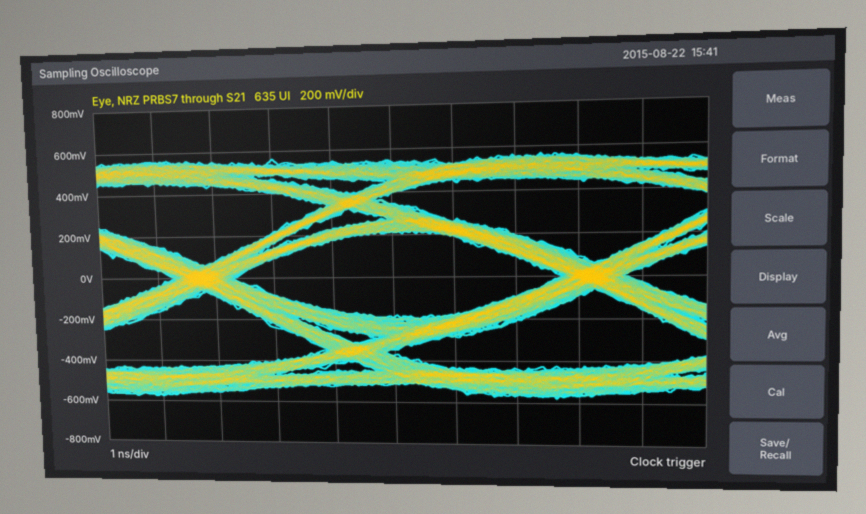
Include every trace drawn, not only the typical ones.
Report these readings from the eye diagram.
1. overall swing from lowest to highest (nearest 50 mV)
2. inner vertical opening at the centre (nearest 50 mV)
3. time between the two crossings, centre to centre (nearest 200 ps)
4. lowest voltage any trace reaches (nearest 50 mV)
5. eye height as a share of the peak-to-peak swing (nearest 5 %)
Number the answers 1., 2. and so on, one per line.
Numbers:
1. 1.15 V
2. 400 mV
3. 6.4 ns
4. -600 mV
5. 35 %
